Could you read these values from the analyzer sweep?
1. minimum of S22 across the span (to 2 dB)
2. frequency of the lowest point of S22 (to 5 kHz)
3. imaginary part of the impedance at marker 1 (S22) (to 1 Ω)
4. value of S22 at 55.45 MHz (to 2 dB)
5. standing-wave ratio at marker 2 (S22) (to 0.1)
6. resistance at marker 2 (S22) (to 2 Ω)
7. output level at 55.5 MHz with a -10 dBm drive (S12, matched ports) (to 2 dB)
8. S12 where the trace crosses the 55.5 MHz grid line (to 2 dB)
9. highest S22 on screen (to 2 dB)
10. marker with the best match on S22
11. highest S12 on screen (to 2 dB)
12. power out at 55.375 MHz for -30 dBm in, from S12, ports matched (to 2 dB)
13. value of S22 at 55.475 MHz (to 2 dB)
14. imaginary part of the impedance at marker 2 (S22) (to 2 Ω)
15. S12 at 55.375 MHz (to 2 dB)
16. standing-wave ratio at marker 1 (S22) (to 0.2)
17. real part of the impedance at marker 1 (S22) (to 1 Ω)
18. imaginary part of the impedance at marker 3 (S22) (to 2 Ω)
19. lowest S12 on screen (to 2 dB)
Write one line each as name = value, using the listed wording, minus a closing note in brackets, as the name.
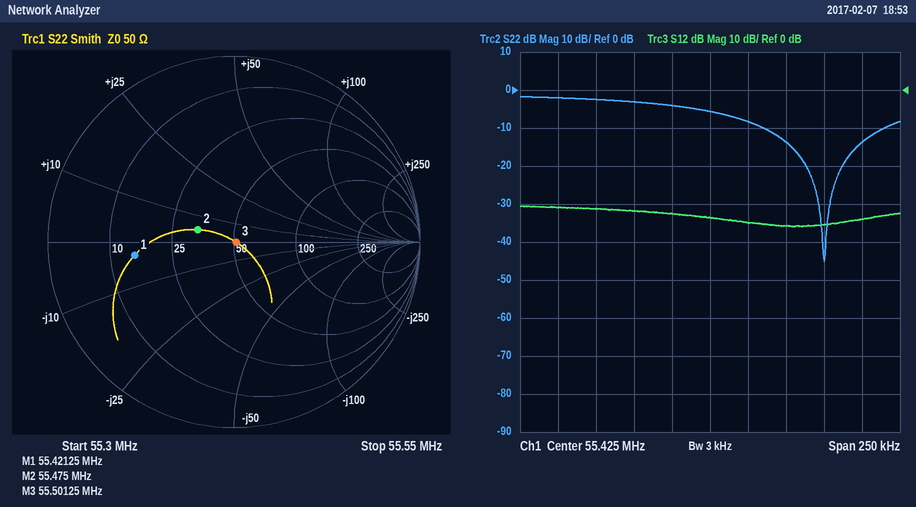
minimum of S22 across the span = -46 dB
frequency of the lowest point of S22 = 55.500 MHz
imaginary part of the impedance at marker 1 (S22) = -3 Ω
value of S22 at 55.45 MHz = -8 dB
standing-wave ratio at marker 2 (S22) = 1.5
resistance at marker 2 (S22) = 34 Ω
output level at 55.5 MHz with a -10 dBm drive (S12, matched ports) = -46 dBm
S12 where the trace crosses the 55.5 MHz grid line = -36 dB
highest S22 on screen = -2 dB
marker with the best match on S22 = marker 3
highest S12 on screen = -30 dB
power out at 55.375 MHz for -30 dBm in, from S12, ports matched = -62 dBm
value of S22 at 55.475 MHz = -14 dB
imaginary part of the impedance at marker 2 (S22) = +4 Ω
S12 at 55.375 MHz = -32 dB
standing-wave ratio at marker 1 (S22) = 3.4
real part of the impedance at marker 1 (S22) = 15 Ω
imaginary part of the impedance at marker 3 (S22) = 0 Ω
lowest S12 on screen = -36 dB
